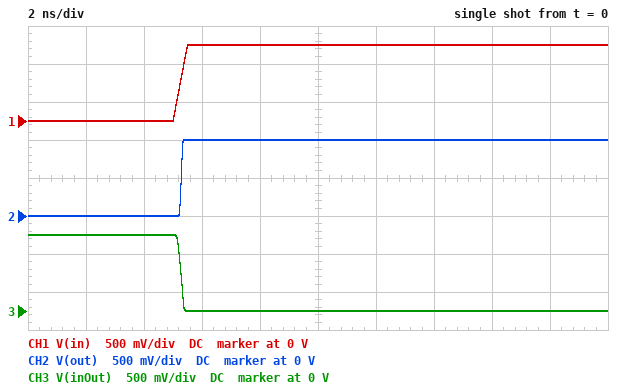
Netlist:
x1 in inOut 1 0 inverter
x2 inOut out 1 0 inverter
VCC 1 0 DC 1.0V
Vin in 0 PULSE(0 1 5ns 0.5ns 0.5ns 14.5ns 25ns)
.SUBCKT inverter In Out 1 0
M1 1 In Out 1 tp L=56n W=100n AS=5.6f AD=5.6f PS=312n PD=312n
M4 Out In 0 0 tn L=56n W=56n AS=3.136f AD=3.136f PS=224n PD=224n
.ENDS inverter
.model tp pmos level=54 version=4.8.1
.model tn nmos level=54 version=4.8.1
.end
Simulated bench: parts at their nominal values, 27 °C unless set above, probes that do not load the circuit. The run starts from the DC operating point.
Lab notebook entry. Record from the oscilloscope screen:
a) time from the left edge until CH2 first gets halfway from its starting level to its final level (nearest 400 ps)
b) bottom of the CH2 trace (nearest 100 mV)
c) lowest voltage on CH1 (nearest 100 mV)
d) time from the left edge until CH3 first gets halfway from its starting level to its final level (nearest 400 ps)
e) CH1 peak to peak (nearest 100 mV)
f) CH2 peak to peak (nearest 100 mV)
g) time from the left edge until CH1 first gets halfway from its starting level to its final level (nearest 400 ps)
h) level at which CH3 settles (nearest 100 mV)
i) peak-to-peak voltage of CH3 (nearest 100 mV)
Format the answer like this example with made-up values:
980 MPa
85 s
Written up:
5.2 ns
0 V
0 V
5.2 ns
1.0 V
1.0 V
5.2 ns
0 V
1.0 V
